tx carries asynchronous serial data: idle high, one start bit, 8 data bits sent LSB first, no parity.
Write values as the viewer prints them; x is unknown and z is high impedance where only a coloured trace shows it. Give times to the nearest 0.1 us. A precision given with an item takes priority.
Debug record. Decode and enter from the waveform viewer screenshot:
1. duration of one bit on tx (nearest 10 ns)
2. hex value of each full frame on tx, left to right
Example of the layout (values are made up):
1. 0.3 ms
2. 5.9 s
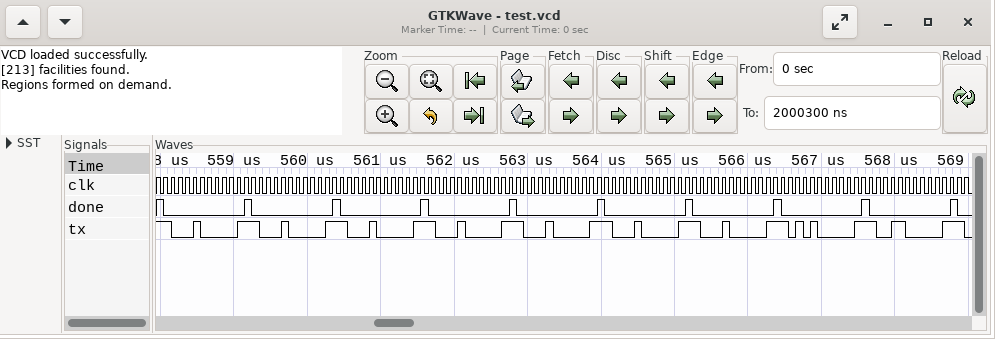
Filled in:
1. 100 ns
2. 04, 04, 04, 04, 04, 04, 04, 05, 06
